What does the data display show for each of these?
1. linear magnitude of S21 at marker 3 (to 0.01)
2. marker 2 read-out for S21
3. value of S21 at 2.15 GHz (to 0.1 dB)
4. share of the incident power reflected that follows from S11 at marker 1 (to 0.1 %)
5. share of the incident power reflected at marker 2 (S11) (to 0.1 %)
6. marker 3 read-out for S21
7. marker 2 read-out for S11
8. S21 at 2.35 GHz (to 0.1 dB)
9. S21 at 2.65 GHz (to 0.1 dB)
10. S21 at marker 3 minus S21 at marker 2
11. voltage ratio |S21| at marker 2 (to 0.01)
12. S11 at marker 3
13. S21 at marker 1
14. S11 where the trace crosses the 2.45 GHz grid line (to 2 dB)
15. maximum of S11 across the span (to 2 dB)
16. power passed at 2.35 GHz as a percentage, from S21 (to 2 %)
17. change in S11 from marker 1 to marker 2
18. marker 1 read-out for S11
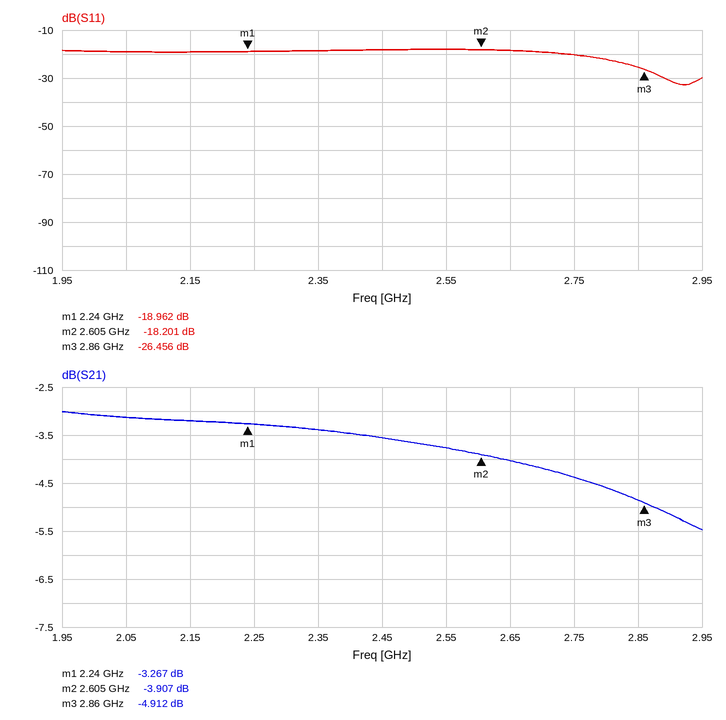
0.57
-3.907 dB
-3.2 dB
1.3 %
1.5 %
-4.912 dB
-18.201 dB
-3.4 dB
-4.0 dB
-1.005 dB
0.64
-26.456 dB
-3.267 dB
-18 dB
-18 dB
46 %
0.761 dB
-18.962 dB
